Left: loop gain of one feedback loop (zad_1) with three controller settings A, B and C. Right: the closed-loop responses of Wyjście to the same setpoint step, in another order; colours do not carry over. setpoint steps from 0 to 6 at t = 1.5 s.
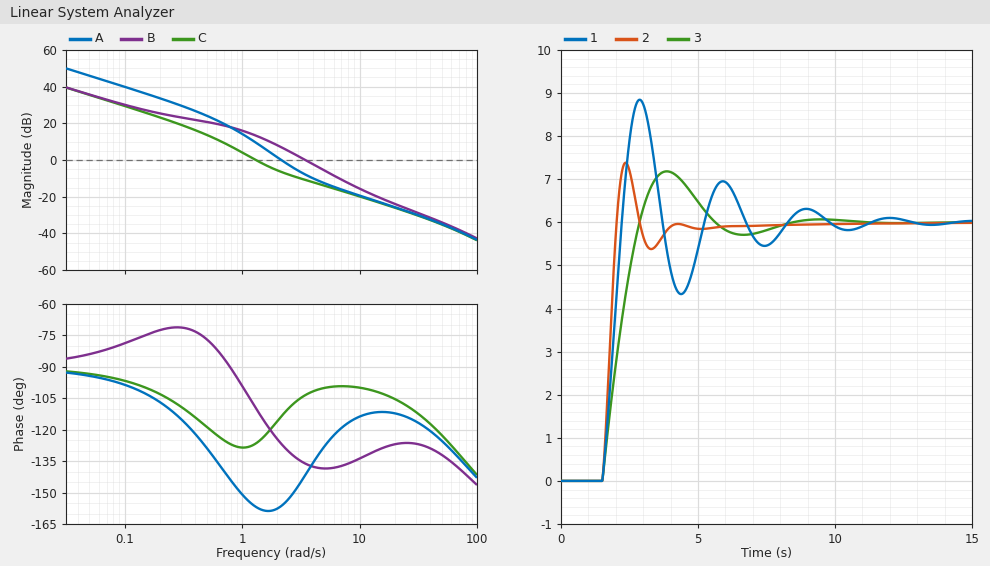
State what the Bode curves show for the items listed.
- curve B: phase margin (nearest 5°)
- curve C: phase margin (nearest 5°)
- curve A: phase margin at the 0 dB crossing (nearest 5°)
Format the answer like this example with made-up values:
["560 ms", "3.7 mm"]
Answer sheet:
["45°", "55°", "25°"]
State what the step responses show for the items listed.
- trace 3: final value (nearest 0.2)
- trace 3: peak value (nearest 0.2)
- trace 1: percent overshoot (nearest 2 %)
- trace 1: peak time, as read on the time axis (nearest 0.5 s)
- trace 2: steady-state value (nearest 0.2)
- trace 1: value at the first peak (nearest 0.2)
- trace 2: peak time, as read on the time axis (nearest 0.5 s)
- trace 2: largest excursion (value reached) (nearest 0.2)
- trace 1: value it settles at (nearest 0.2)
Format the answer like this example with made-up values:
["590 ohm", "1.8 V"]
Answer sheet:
["6.0", "7.2", "48 %", "3.0 s", "6.0", "8.8", "2.5 s", "7.4", "6.0"]
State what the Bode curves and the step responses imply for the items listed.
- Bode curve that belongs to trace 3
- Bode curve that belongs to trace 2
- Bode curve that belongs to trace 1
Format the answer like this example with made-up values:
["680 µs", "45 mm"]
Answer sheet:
["C", "B", "A"]
